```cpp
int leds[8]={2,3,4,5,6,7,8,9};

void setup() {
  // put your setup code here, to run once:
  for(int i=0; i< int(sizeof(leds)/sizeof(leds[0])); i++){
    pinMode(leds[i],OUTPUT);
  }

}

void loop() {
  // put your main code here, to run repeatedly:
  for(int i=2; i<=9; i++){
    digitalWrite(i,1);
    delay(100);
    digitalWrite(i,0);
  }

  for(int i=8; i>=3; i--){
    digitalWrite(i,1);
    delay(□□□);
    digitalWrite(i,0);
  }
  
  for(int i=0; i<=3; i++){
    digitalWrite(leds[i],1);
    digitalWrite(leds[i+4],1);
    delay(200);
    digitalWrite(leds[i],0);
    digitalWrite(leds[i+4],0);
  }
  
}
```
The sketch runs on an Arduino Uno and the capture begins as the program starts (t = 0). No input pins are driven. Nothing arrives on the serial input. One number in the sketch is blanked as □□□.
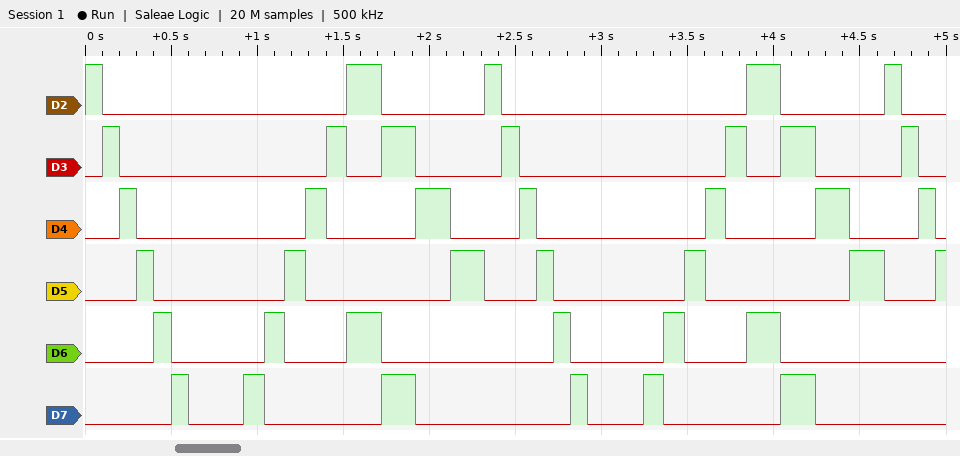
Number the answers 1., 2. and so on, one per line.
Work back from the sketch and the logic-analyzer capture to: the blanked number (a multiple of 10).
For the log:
1. 120
